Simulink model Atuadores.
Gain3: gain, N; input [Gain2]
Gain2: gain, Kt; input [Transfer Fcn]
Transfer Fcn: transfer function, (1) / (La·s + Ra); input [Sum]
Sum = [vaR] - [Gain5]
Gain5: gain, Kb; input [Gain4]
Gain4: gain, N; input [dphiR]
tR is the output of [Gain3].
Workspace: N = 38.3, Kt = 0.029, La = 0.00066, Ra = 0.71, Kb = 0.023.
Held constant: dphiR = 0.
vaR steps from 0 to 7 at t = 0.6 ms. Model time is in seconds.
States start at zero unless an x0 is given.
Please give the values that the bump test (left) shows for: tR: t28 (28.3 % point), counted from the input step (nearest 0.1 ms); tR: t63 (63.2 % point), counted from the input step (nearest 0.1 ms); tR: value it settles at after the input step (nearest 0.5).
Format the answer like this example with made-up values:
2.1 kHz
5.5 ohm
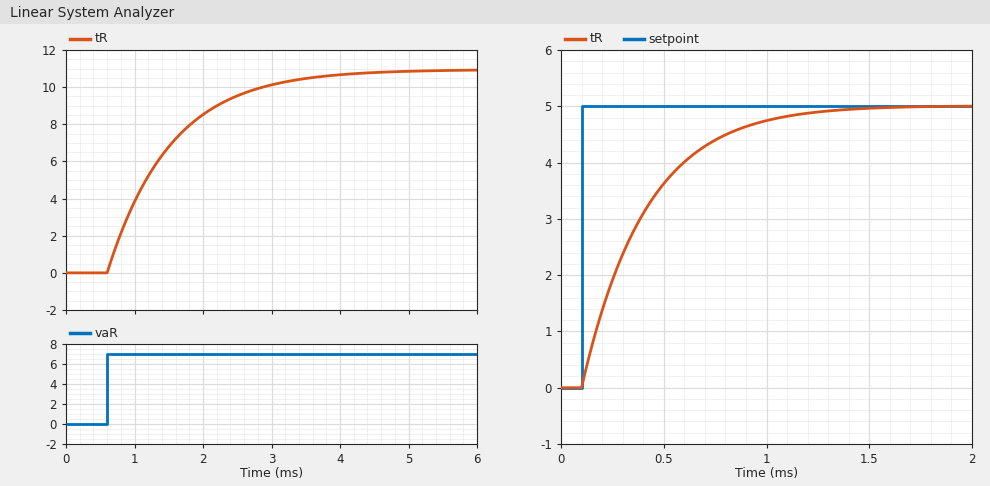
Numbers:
0.3 ms
0.9 ms
11.0
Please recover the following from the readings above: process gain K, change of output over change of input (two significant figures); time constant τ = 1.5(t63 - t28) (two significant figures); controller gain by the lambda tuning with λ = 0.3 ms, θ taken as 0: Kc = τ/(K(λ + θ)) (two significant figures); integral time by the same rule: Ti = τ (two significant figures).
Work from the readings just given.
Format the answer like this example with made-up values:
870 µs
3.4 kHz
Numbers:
1.6
0.90 ms
1.9
0.90 ms
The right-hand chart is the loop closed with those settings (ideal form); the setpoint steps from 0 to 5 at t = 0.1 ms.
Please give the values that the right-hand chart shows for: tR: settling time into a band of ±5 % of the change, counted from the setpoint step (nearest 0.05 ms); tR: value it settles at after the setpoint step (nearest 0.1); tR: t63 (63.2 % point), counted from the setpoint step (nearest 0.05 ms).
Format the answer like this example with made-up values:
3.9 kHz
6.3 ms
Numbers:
0.90 ms
5.0
0.30 ms
